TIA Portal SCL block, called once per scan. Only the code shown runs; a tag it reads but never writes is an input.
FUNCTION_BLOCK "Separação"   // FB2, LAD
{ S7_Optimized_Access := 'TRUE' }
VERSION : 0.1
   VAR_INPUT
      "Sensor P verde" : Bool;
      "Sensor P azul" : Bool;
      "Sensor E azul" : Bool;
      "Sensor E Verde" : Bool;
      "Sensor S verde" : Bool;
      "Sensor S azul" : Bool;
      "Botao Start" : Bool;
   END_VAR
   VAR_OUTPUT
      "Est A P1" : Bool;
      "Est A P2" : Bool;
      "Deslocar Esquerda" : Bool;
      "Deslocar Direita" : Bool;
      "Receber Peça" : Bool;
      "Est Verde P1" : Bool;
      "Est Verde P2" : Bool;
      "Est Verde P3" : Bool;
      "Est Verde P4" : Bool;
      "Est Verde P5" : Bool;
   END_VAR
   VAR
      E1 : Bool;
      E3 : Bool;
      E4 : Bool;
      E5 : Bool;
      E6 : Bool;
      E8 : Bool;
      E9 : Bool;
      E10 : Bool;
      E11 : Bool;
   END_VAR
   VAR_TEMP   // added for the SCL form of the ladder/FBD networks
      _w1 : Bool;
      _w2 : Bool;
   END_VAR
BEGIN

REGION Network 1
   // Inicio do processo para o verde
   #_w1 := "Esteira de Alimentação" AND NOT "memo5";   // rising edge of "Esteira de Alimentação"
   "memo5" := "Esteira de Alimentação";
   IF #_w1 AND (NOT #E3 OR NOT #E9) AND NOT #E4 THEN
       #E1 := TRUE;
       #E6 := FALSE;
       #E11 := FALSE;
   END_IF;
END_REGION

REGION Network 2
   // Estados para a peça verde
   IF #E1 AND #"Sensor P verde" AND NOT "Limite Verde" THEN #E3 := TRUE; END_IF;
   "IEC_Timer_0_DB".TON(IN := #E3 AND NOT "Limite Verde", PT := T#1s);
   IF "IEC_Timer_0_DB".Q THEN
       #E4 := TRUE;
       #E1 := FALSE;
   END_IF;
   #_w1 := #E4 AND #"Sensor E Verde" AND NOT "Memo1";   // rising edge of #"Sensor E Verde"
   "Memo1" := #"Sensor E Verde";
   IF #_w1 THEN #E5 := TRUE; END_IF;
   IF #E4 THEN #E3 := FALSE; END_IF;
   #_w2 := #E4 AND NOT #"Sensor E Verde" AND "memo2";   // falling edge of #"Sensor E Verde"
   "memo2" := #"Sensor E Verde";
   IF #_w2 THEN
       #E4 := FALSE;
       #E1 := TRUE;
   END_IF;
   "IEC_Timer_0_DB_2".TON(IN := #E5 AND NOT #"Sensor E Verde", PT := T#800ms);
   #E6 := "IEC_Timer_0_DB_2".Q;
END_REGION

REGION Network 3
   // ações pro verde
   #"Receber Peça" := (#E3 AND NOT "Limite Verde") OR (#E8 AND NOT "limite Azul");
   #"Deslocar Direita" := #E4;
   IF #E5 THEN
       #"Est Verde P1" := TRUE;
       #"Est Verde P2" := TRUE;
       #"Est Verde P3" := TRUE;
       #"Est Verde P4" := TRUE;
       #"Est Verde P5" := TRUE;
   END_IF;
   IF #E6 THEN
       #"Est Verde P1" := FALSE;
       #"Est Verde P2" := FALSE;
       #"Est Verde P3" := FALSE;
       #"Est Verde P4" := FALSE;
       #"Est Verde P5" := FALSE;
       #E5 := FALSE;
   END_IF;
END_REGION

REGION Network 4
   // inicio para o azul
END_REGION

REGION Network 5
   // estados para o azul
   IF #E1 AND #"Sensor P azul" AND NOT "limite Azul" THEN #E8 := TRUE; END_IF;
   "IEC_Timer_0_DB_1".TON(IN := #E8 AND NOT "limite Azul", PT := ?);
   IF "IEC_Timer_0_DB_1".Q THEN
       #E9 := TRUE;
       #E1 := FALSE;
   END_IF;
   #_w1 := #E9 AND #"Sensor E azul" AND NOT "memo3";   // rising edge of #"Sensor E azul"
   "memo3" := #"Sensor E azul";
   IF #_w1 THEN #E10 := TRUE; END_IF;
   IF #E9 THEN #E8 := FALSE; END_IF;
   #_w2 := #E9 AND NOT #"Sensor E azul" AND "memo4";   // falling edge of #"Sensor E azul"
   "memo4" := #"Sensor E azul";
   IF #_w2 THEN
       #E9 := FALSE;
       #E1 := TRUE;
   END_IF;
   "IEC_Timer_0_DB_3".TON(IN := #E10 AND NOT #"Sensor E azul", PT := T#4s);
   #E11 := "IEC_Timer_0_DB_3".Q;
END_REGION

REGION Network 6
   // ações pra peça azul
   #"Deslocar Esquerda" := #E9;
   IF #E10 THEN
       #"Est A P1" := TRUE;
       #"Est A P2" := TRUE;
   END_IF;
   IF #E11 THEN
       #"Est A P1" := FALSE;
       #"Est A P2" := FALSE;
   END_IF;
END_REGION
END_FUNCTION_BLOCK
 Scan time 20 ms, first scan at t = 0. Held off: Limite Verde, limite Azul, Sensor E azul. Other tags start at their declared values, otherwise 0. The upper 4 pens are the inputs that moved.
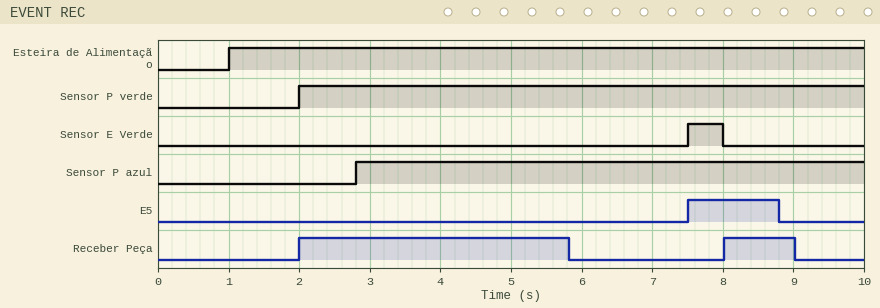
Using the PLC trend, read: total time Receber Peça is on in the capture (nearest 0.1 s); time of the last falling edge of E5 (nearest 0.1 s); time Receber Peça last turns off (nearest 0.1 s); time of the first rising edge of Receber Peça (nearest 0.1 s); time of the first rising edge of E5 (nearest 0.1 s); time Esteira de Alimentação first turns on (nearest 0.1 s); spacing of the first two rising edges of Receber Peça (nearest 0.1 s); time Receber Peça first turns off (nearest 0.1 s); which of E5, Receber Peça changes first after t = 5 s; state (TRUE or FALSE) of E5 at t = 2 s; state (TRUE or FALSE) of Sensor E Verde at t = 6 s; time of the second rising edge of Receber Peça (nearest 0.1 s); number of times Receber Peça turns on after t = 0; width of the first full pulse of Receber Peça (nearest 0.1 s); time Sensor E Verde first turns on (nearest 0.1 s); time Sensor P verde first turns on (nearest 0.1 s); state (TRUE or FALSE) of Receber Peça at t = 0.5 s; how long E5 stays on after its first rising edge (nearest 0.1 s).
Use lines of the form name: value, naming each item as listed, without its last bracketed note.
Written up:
total time Receber Peça is on in the capture: 4.8 s
time of the last falling edge of E5: 8.8 s
time Receber Peça last turns off: 9.0 s
time of the first rising edge of Receber Peça: 2.0 s
time of the first rising edge of E5: 7.5 s
time Esteira de Alimentação first turns on: 1.0 s
spacing of the first two rising edges of Receber Peça: 6.0 s
time Receber Peça first turns off: 5.8 s
which of E5, Receber Peça changes first after t = 5 s: Receber Peça
state (TRUE or FALSE) of E5 at t = 2 s: FALSE
state (TRUE or FALSE) of Sensor E Verde at t = 6 s: FALSE
time of the second rising edge of Receber Peça: 8.0 s
number of times Receber Peça turns on after t = 0: 2
width of the first full pulse of Receber Peça: 3.8 s
time Sensor E Verde first turns on: 7.5 s
time Sensor P verde first turns on: 2.0 s
state (TRUE or FALSE) of Receber Peça at t = 0.5 s: FALSE
how long E5 stays on after its first rising edge: 1.3 s
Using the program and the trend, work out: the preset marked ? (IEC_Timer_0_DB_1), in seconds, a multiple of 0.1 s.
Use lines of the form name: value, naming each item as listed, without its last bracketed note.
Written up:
the preset marked ? (IEC_Timer_0_DB_1), in seconds, a multiple of 0.1 s: 3.0 s
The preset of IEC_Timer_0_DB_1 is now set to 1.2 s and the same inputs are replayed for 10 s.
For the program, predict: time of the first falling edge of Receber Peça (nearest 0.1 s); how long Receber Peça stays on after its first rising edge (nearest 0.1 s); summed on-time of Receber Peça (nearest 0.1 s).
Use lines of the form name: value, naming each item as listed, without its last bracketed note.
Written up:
time of the first falling edge of Receber Peça: 4.0 s
how long Receber Peça stays on after its first rising edge: 2.0 s
summed on-time of Receber Peça: 3.0 s
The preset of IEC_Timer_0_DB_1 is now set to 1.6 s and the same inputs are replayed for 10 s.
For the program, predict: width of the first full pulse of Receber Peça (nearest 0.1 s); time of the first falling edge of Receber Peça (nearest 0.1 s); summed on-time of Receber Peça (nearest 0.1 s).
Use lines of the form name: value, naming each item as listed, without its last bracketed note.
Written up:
width of the first full pulse of Receber Peça: 2.4 s
time of the first falling edge of Receber Peça: 4.4 s
summed on-time of Receber Peça: 3.4 s
